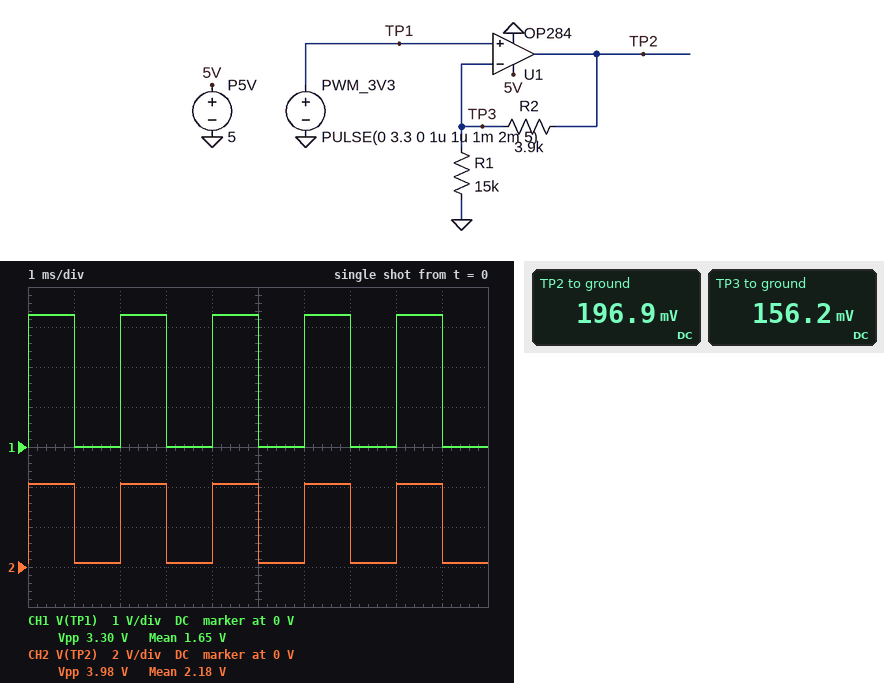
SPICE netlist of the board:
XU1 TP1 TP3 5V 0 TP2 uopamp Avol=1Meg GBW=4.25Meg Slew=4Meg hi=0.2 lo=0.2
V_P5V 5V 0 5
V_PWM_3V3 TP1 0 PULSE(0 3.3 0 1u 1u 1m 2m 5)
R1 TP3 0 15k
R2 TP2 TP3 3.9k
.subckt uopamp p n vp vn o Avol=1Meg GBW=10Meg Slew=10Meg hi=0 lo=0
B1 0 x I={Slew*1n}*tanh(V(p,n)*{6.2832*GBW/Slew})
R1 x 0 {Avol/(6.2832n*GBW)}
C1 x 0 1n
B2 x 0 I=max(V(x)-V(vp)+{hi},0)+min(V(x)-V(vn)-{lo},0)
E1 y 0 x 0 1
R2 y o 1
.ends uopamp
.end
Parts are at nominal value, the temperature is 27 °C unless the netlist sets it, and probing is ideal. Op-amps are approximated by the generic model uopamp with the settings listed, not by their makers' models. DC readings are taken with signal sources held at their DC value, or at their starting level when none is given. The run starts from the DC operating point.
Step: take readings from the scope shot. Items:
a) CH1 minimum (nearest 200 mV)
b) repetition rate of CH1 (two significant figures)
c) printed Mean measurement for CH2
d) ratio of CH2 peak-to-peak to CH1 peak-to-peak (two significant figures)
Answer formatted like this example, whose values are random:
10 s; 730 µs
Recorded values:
0 V; 500 Hz; 2.18 V; 1.2
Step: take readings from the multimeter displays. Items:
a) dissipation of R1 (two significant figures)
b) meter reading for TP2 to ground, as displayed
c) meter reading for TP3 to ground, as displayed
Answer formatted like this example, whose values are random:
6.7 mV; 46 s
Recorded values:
1.6 µW; 196.9 mV; 156.2 mV
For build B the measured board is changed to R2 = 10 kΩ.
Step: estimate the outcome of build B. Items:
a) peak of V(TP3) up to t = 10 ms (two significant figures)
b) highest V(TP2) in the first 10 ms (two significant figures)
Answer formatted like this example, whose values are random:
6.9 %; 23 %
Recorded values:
2.9 V; 4.8 V
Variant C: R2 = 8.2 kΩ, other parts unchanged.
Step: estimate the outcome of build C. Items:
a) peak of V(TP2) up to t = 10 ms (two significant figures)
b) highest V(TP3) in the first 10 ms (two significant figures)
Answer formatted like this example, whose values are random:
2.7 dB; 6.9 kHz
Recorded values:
4.8 V; 3.1 V
